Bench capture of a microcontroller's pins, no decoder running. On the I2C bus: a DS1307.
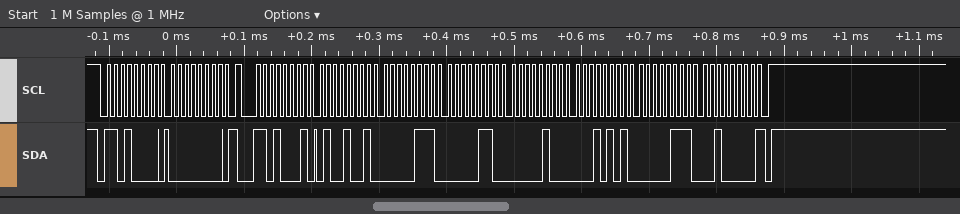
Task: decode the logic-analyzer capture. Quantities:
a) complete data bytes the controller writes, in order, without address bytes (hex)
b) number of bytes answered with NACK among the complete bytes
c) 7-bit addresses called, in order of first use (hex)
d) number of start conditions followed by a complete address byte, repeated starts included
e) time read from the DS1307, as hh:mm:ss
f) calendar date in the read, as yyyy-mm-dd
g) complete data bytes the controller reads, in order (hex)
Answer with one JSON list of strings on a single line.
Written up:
["00", "1", "0x68", "2", "06:07:49", "2020-07-15", "49 07 06 04 15 07 20"]
